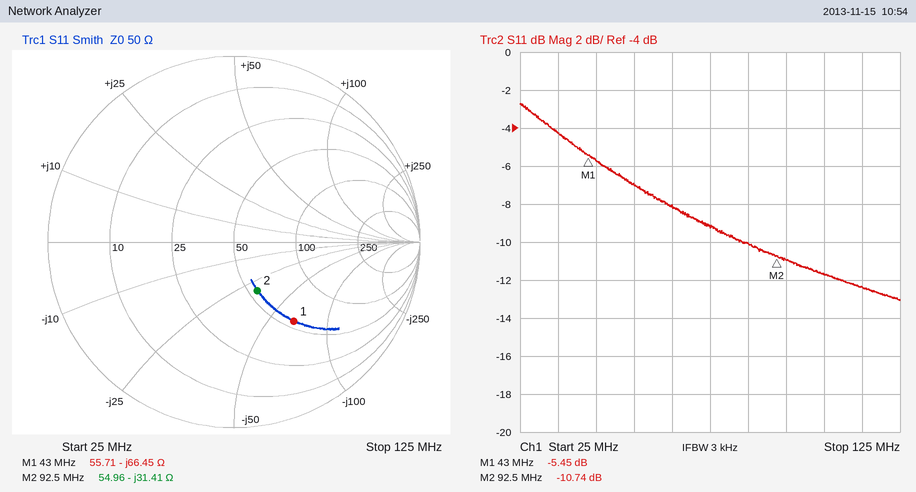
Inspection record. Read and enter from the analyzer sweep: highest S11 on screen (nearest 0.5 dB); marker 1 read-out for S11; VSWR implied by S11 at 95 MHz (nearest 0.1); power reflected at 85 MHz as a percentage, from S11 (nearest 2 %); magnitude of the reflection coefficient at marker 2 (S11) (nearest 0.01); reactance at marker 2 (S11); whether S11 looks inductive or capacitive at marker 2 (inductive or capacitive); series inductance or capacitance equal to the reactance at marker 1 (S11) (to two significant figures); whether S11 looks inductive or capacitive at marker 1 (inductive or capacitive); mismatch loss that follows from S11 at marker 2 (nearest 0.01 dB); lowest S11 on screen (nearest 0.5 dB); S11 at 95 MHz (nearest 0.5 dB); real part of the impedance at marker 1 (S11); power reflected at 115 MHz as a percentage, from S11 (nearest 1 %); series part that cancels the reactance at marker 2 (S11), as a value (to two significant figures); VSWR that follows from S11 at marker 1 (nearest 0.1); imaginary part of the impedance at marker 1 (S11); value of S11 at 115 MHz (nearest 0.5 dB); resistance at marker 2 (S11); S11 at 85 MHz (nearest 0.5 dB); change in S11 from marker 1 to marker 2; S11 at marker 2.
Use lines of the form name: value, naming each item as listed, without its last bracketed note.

highest S11 on screen: -2.5 dB
marker 1 read-out for S11: -5.45 dB
VSWR implied by S11 at 95 MHz: 1.8
power reflected at 85 MHz as a percentage, from S11: 10 %
magnitude of the reflection coefficient at marker 2 (S11): 0.29
reactance at marker 2: -31.41 Ω
whether S11 looks inductive or capacitive at marker 2: capacitive
series inductance or capacitance equal to the reactance at marker 1 (S11): 56 pF
whether S11 looks inductive or capacitive at marker 1: capacitive
mismatch loss that follows from S11 at marker 2: 0.38 dB
lowest S11 on screen: -13.0 dB
S11 at 95 MHz: -11.0 dB
real part of the impedance at marker 1: 55.71 Ω
power reflected at 115 MHz as a percentage, from S11: 6 %
series part that cancels the reactance at marker 2 (S11), as a value: 54 nH
VSWR that follows from S11 at marker 1: 3.3
imaginary part of the impedance at marker 1: -66.45 Ω
value of S11 at 115 MHz: -12.5 dB
resistance at marker 2: 54.96 Ω
S11 at 85 MHz: -10.0 dB
change in S11 from marker 1 to marker 2: -5.29 dB
S11 at marker 2: -10.74 dB
